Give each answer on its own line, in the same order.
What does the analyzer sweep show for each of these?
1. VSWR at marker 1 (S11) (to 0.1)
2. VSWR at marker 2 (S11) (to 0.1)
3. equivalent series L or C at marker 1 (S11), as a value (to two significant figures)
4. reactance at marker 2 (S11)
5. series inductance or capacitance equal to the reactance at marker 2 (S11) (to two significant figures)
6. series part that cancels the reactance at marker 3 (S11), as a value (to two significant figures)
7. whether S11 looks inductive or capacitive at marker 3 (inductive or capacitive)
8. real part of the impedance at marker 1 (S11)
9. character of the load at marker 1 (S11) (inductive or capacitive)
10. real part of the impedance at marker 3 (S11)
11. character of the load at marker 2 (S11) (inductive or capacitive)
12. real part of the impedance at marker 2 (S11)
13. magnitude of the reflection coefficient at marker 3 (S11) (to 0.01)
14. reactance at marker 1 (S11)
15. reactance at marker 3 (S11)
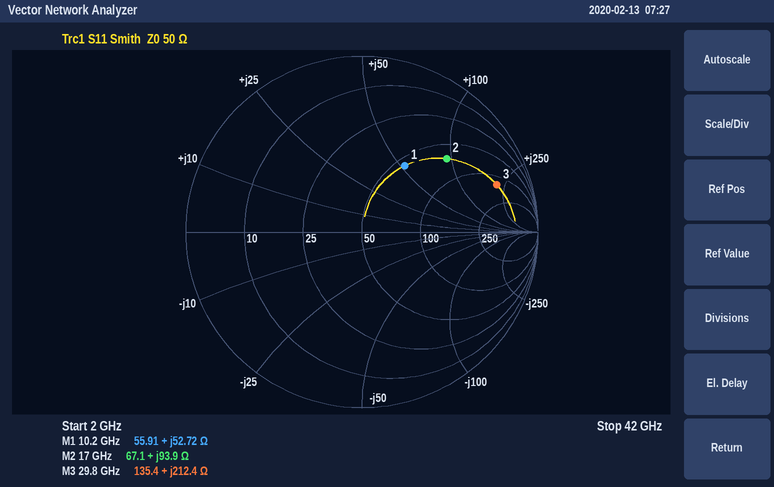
2.6
4.5
820 pH
+93.9 Ω
880 pH
25 fF
inductive
55.91 Ω
inductive
135.4 Ω
inductive
67.1 Ω
0.81
+52.72 Ω
+212.4 Ω
